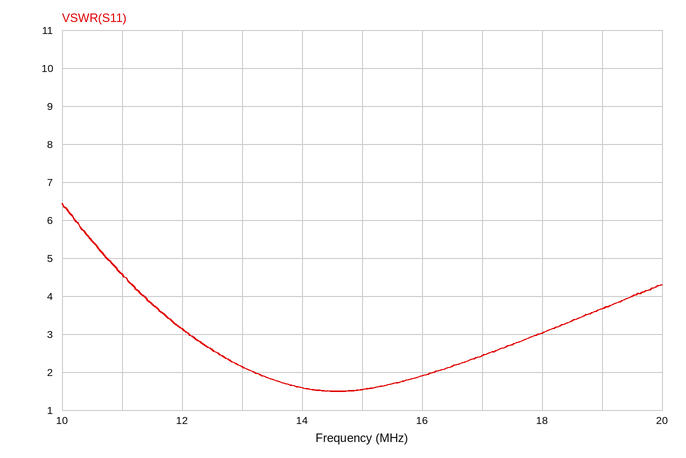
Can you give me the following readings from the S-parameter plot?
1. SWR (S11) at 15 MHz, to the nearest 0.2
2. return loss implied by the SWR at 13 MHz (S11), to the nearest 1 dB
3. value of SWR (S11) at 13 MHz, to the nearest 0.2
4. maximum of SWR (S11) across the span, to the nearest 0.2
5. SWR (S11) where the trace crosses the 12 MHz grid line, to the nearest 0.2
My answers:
1.6
9 dB
2.2
6.4
3.2
